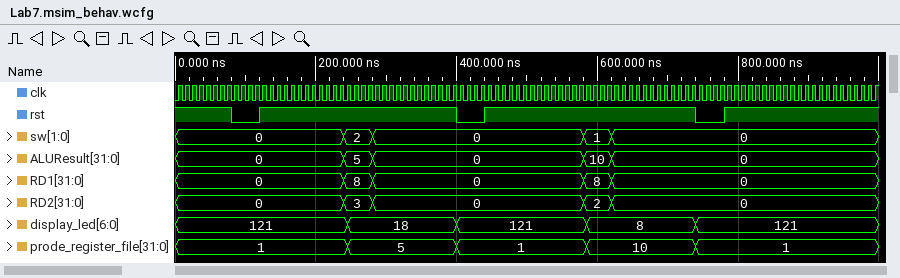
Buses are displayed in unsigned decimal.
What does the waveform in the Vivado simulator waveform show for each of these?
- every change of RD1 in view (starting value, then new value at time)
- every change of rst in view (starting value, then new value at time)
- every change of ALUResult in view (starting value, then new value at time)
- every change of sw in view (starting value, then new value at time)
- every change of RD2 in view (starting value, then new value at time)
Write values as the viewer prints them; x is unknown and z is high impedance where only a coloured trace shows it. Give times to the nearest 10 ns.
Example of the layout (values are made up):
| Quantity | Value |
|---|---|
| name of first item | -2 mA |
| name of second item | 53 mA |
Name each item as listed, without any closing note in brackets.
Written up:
| Quantity | Value |
|---|---|
| every change of RD1 in view | 0, 8 at 240 ns, 0 at 280 ns, 8 at 580 ns, 0 at 620 ns |
| every change of rst in view | 1, 0 at 80 ns, 1 at 120 ns, 0 at 400 ns, 1 at 440 ns, 0 at 740 ns, 1 at 780 ns |
| every change of ALUResult in view | 0, 5 at 240 ns, 0 at 280 ns, 10 at 580 ns, 0 at 620 ns |
| every change of sw in view | 0, 2 at 240 ns, 0 at 280 ns, 1 at 580 ns, 0 at 620 ns |
| every change of RD2 in view | 0, 3 at 240 ns, 0 at 280 ns, 2 at 580 ns, 0 at 620 ns |
